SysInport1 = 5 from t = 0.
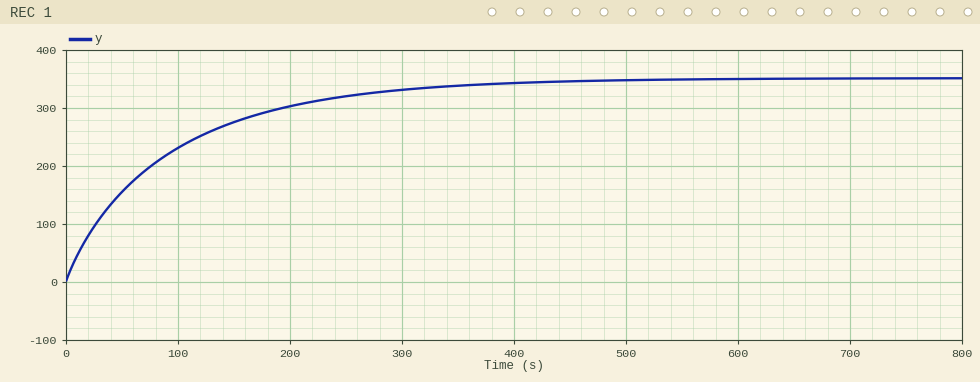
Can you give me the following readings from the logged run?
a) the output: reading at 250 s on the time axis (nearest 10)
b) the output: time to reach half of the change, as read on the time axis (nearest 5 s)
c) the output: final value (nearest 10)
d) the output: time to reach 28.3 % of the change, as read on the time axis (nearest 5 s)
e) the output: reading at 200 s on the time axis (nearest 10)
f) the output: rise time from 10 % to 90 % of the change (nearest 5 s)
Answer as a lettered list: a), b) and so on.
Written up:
a) 320
b) 60 s
c) 350
d) 25 s
e) 300
f) 230 s
